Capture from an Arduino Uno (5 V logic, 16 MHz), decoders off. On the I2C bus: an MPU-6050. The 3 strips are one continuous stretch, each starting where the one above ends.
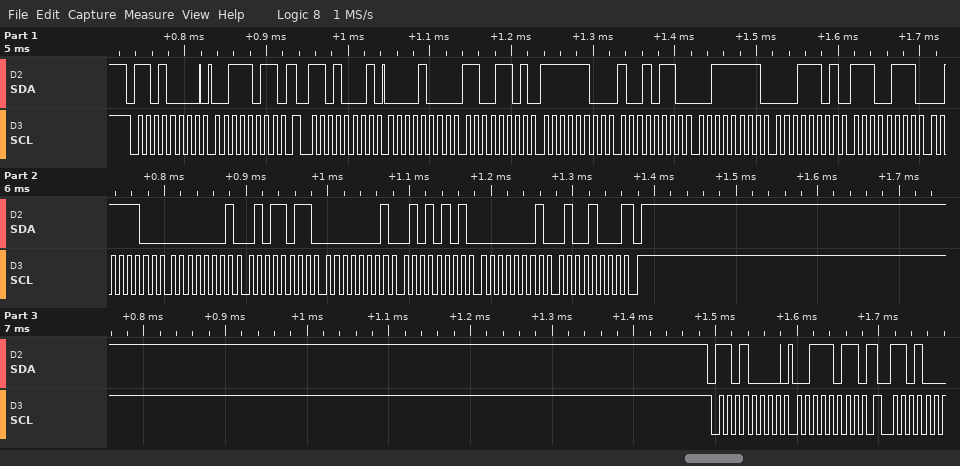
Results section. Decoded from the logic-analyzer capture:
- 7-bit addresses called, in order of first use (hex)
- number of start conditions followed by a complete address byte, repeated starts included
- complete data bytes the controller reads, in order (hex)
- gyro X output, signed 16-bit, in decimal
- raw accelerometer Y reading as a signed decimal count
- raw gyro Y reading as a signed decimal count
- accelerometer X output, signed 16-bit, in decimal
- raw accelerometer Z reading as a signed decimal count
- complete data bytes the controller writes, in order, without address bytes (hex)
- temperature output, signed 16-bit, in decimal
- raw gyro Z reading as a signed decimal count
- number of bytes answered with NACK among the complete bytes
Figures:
0x68
3
08 CD FC 96 3F 1D E7 3C 01 5B 01 55 01 48
347
-874
341
2253
16157
3B 3B
-6340
328
1
